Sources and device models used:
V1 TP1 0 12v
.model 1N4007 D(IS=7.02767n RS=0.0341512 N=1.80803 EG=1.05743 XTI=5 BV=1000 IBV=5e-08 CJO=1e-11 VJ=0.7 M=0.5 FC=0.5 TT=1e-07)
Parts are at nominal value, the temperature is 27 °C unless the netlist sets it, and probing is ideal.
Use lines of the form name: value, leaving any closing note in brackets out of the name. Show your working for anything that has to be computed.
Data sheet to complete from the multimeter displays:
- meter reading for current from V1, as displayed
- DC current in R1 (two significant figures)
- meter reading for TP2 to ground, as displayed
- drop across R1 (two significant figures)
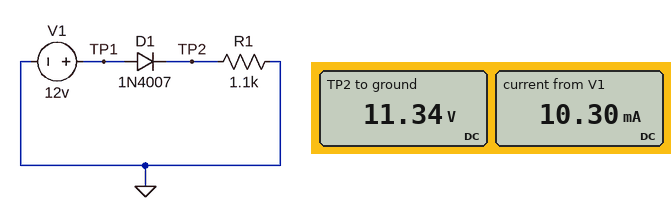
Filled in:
meter reading for current from V1, as displayed: 10.30 mA
DC current in R1: (11.34 V) / 1.1 kΩ = 10 mA
meter reading for TP2 to ground, as displayed: 11.34 V
drop across R1: 11.34 V = 11 V
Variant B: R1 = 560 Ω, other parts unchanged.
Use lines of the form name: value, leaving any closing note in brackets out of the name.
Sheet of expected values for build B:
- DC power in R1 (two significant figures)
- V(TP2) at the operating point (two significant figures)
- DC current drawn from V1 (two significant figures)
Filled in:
DC power in R1: 230 mW
V(TP2) at the operating point: 11 V
DC current drawn from V1: 20 mA
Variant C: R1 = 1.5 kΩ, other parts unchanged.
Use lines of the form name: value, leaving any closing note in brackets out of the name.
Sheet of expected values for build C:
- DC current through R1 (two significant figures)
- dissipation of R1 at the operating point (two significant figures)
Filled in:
DC current through R1: 7.6 mA
dissipation of R1 at the operating point: 86 mW
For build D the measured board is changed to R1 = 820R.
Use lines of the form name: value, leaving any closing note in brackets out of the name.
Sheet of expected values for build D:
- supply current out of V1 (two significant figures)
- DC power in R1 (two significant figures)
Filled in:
supply current out of V1: 14 mA
DC power in R1: 160 mW
